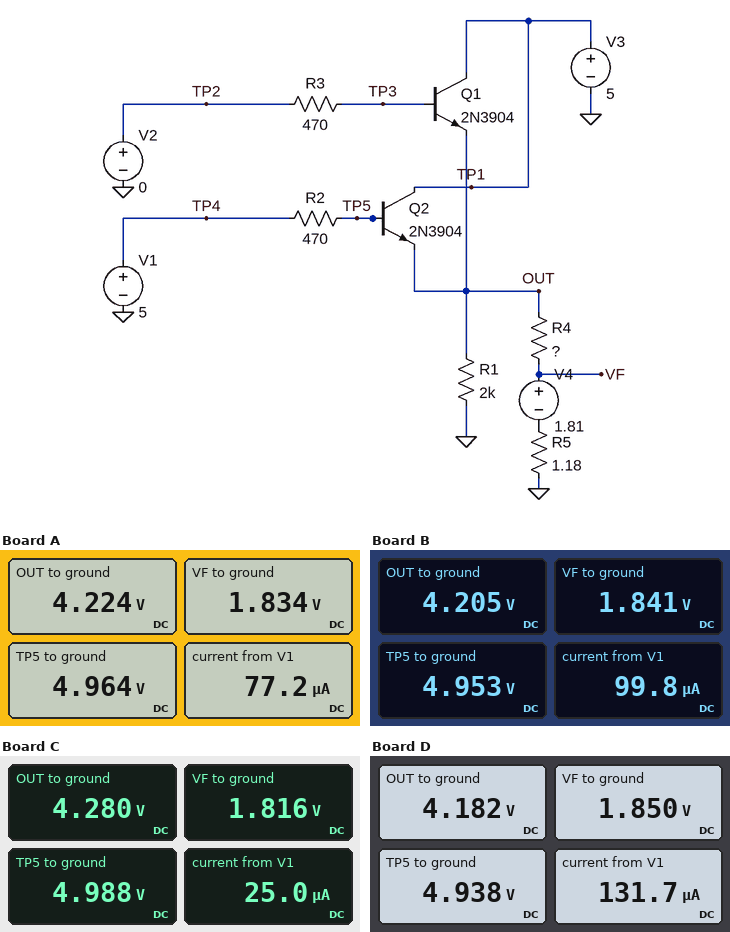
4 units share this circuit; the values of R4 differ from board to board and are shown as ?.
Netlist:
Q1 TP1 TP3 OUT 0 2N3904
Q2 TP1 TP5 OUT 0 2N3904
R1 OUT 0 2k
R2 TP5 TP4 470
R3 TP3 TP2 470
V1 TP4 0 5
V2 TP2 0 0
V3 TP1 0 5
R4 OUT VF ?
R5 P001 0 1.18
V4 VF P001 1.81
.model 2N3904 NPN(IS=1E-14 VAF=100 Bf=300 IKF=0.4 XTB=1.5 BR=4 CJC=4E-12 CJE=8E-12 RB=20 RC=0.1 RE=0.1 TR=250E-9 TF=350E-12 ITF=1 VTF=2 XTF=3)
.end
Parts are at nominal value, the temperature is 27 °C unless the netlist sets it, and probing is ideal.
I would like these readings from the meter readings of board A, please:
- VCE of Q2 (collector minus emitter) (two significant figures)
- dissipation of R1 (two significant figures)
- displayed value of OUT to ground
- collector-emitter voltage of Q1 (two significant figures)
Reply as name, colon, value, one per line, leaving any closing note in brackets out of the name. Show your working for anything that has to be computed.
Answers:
VCE of Q2 (collector minus emitter): 5 V - 4.224 V = 780 mV
dissipation of R1: (4.224 V)^2 / 2 kΩ = 8.9 mW
displayed value of OUT to ground: 4.224 V
collector-emitter voltage of Q1: 5 V - 4.224 V = 780 mV
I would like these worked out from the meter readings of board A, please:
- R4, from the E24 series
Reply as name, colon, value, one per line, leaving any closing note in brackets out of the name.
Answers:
R4, from the E24 series: 120 Ω
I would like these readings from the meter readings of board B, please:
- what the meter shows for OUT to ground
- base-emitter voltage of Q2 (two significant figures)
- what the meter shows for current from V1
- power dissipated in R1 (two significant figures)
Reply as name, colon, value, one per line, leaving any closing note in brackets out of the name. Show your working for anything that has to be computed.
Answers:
what the meter shows for OUT to ground: 4.205 V
base-emitter voltage of Q2: 4.953 V - 4.205 V = 750 mV
what the meter shows for current from V1: 99.8 µA
power dissipated in R1: (4.205 V)^2 / 2 kΩ = 8.8 mW
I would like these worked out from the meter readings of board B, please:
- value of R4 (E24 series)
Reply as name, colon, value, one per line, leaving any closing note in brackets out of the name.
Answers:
value of R4: 91 Ω
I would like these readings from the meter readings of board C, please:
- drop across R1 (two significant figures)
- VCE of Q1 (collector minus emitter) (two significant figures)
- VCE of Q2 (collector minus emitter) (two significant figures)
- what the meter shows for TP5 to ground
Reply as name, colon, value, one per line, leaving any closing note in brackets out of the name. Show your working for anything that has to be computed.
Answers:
drop across R1: 4.28 V = 4.3 V
VCE of Q1 (collector minus emitter): 5 V - 4.28 V = 720 mV
VCE of Q2 (collector minus emitter): 5 V - 4.28 V = 720 mV
what the meter shows for TP5 to ground: 4.988 V
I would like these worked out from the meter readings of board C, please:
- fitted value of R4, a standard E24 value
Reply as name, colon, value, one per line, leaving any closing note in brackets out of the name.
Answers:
fitted value of R4, a standard E24 value: 470 Ω
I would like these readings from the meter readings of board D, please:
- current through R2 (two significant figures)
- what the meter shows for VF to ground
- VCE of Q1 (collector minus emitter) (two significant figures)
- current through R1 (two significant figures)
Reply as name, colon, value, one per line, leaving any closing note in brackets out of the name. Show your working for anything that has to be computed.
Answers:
current through R2: (5 V - 4.938 V) / 470 Ω = 130 µA
what the meter shows for VF to ground: 1.850 V
VCE of Q1 (collector minus emitter): 5 V - 4.182 V = 820 mV
current through R1: (4.182 V) / 2 kΩ = 2.1 mA
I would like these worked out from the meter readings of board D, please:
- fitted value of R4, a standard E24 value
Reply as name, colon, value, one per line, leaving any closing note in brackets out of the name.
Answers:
fitted value of R4, a standard E24 value: 68 Ω
